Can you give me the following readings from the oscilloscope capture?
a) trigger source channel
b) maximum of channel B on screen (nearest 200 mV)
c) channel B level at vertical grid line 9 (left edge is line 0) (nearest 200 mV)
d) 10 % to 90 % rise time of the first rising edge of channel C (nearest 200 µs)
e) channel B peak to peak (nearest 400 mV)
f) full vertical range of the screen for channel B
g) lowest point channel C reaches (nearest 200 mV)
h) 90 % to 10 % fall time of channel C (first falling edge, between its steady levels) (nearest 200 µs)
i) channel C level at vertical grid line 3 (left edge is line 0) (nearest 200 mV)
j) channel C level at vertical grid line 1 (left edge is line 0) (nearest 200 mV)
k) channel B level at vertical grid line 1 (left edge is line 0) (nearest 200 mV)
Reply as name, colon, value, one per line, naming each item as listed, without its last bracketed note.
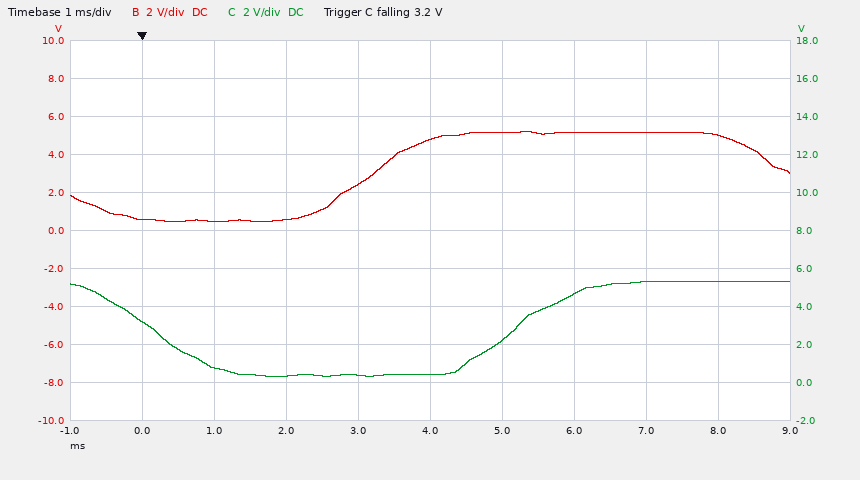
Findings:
trigger source channel: channel C
maximum of channel B on screen: 5.2 V
channel B level at vertical grid line 9 (left edge is line 0): 5.0 V
10 % to 90 % rise time of the first rising edge of channel C: 1.6 ms
channel B peak to peak: 4.8 V
full vertical range of the screen for channel B: 20 V
lowest point channel C reaches: 400 mV
90 % to 10 % fall time of channel C (first falling edge, between its steady levels): 1.6 ms
channel C level at vertical grid line 3 (left edge is line 0): 400 mV
channel C level at vertical grid line 1 (left edge is line 0): 3.2 V
channel B level at vertical grid line 1 (left edge is line 0): 600 mV
